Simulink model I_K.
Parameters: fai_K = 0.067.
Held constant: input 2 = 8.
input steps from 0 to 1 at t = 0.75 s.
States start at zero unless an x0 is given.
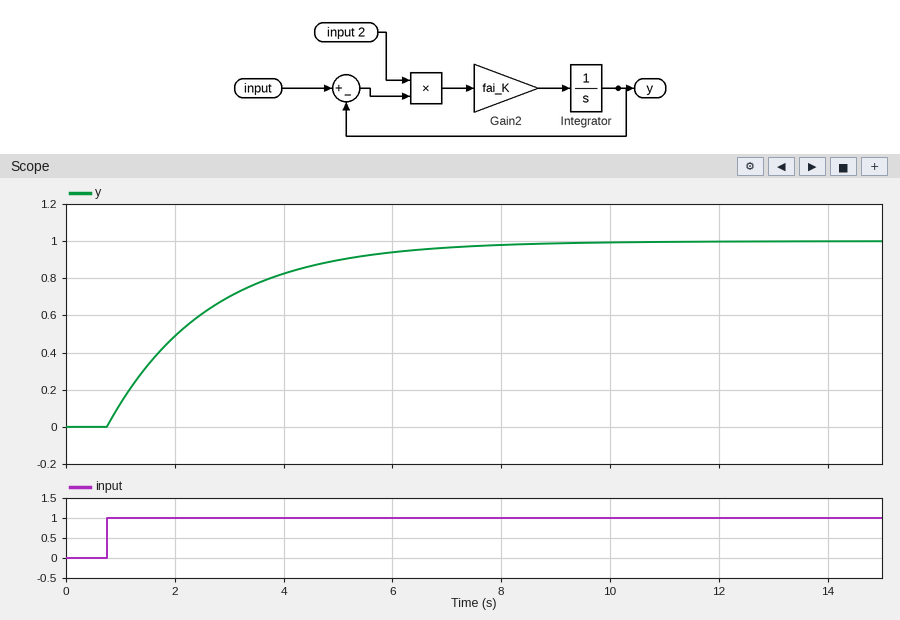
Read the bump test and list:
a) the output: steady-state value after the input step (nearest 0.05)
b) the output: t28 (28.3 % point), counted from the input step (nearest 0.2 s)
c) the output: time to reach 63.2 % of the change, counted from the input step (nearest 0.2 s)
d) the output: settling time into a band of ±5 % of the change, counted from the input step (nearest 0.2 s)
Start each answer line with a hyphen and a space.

- 1.00
- 0.6 s
- 1.8 s
- 5.6 s
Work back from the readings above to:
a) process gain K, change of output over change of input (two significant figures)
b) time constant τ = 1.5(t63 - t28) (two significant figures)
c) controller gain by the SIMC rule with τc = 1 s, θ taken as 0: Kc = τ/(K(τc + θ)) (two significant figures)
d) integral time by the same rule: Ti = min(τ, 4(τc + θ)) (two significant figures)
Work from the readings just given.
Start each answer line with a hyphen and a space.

- 1.0
- 1.8 s
- 1.8
- 1.8 s
